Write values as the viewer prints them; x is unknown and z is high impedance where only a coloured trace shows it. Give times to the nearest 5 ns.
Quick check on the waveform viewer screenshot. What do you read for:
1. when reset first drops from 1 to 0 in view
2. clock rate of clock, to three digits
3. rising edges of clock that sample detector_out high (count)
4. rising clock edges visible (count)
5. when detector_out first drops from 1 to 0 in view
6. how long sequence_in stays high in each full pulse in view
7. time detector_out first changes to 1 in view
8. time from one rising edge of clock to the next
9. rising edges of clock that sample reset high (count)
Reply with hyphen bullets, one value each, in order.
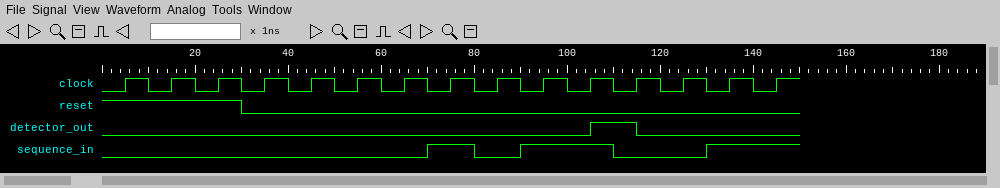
- 30 ns
- 100 MHz
- 1
- 15
- 115 ns
- 10 ns, 20 ns
- 105 ns
- 10 ns
- 3
